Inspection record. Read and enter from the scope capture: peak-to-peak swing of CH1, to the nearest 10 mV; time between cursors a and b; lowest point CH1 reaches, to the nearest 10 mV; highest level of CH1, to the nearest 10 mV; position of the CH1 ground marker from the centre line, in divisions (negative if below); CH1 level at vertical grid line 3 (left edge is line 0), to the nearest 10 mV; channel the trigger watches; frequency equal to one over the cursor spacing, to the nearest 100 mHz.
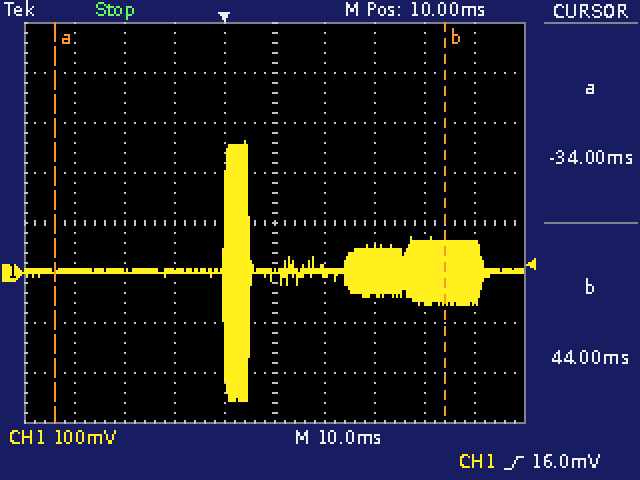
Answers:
520 mV
78 ms
-260 mV
260 mV
-1.0 div
0 mV
CH1
12.8 Hz
